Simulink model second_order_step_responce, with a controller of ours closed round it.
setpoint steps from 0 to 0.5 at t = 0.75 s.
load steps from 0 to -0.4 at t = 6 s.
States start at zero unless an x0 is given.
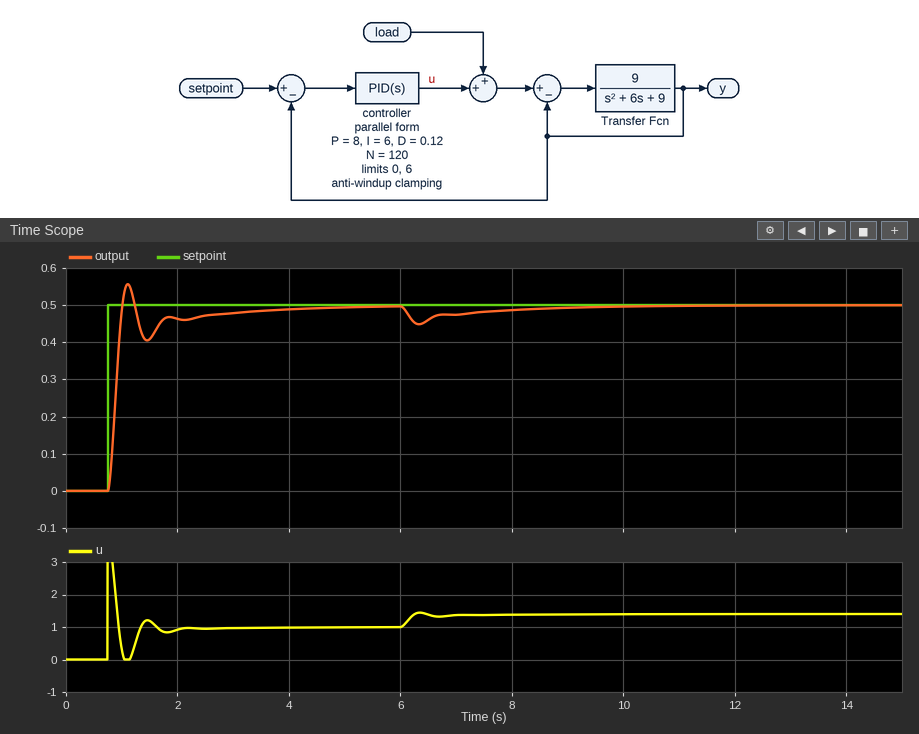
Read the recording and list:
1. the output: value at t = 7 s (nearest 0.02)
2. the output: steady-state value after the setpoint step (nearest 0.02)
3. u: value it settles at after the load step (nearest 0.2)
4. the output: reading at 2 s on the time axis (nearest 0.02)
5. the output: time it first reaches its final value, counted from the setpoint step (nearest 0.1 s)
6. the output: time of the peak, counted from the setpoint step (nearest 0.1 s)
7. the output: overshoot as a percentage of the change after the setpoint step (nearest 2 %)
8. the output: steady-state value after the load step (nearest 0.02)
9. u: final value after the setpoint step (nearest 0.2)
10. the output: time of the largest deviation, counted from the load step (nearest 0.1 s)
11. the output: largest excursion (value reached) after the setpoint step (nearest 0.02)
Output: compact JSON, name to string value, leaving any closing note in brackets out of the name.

{"the output: value at t = 7 s": "0.48", "the output: steady-state value after the setpoint step": "0.50", "u: value it settles at after the load step": "1.4", "the output: reading at 2 s on the time axis": "0.46", "the output: time it first reaches its final value, counted from the setpoint step": "0.3 s", "the output: time of the peak, counted from the setpoint step": "0.4 s", "the output: overshoot as a percentage of the change after the setpoint step": "12 %", "the output: steady-state value after the load step": "0.50", "u: final value after the setpoint step": "1.0", "the output: time of the largest deviation, counted from the load step": "0.3 s", "the output: largest excursion (value reached) after the setpoint step": "0.56"}
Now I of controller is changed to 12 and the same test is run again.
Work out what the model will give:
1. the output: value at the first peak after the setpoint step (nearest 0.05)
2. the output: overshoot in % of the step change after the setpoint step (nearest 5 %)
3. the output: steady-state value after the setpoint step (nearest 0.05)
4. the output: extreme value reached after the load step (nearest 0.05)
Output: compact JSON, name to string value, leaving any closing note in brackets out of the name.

{"the output: value at the first peak after the setpoint step": "0.60", "the output: overshoot in % of the step change after the setpoint step": "20 %", "the output: steady-state value after the setpoint step": "0.50", "the output: extreme value reached after the load step": "0.45"}
